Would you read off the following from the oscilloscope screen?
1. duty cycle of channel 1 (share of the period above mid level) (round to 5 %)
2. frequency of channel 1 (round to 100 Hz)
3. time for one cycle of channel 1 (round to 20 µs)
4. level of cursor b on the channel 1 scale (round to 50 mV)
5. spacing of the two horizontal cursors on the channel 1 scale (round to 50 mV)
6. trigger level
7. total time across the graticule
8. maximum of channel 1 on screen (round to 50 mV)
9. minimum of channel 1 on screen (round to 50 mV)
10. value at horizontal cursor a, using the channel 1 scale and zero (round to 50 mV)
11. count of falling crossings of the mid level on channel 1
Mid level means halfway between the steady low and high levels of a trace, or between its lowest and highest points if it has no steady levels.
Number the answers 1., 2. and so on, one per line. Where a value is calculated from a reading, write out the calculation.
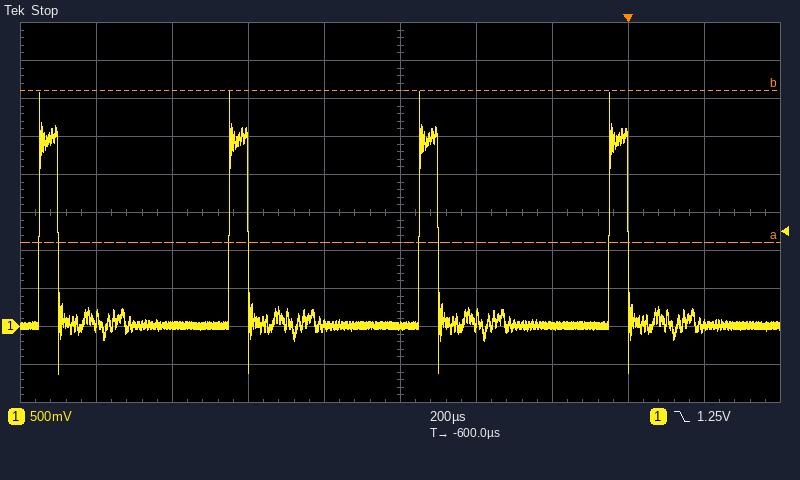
1. 10 %
2. 1 / 500 µs ≈ 2.0 kHz
3. 500 µs
4. 3.10 V
5. 2.00 V
6. 1.25 V
7. 2 ms
8. 3.10 V
9. -650 mV
10. 1.10 V
11. 4
